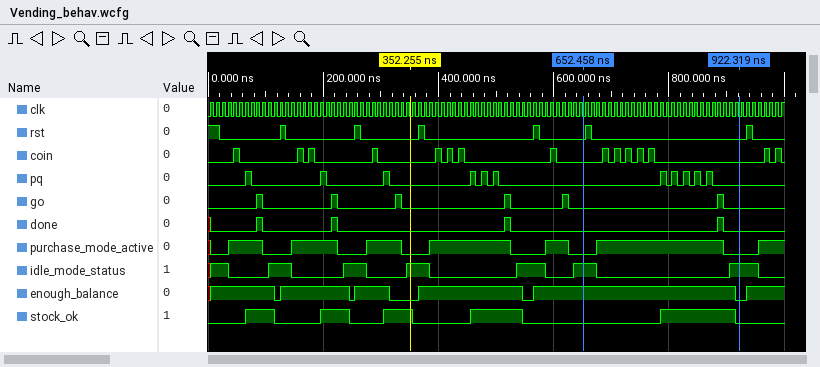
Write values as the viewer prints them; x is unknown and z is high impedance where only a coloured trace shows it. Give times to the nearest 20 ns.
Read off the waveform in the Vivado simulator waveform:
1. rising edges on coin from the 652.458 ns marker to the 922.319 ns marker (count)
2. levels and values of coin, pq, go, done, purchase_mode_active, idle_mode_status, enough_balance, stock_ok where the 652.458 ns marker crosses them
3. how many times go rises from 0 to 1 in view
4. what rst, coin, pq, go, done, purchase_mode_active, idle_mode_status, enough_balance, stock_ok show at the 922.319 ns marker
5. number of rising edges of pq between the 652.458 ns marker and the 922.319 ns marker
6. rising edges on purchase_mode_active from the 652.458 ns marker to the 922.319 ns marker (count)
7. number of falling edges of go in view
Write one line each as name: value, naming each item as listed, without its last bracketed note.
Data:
rising edges on coin from the 652.458 ns marker to the 922.319 ns marker: 5
levels and values of coin, pq, go, done, purchase_mode_active, idle_mode_status, enough_balance, stock_ok where the 652.458 ns marker crosses them: coin=0, pq=0, go=0, done=0, purchase_mode_active=0, idle_mode_status=1, enough_balance=1, stock_ok=0
how many times go rises from 0 to 1 in view: 6
what rst, coin, pq, go, done, purchase_mode_active, idle_mode_status, enough_balance, stock_ok show at the 922.319 ns marker: rst=0, coin=0, pq=0, go=0, done=0, purchase_mode_active=0, idle_mode_status=1, enough_balance=0, stock_ok=0
number of rising edges of pq between the 652.458 ns marker and the 922.319 ns marker: 5
rising edges on purchase_mode_active from the 652.458 ns marker to the 922.319 ns marker: 1
number of falling edges of go in view: 6
